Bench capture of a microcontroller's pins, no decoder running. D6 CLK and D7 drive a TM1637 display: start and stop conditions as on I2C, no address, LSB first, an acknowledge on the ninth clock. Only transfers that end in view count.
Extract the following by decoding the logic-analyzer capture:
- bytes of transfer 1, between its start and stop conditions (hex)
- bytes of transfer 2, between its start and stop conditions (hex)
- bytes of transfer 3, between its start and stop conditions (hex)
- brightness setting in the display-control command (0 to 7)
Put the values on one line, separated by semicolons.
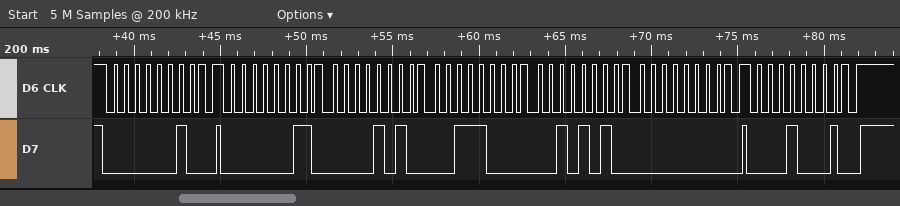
40; C0 50 1C 54 00; 88; 0
